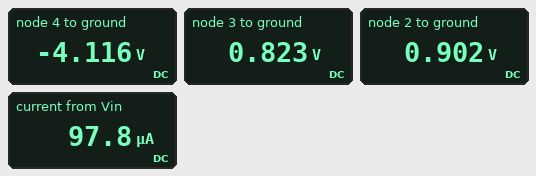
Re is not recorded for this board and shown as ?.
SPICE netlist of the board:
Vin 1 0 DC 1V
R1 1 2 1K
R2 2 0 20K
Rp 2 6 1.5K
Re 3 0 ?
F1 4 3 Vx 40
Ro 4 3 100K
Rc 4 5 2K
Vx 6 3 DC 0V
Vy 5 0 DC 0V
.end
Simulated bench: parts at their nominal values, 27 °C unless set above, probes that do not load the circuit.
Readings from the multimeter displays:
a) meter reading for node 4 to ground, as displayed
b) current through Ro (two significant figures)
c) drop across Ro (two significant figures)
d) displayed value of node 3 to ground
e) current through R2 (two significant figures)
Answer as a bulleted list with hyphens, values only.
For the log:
- -4.116 V
- 49 µA
- 4.9 V
- 0.823 V
- 45 µA
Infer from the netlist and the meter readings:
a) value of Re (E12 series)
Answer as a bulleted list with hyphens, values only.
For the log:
- 390 Ω
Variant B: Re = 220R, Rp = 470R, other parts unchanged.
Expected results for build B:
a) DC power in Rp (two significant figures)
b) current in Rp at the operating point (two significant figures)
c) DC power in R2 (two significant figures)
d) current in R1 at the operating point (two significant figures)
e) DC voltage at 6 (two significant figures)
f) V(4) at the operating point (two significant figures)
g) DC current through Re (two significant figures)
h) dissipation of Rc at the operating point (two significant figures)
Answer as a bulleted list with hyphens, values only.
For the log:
- 4.1 µW
- 93 µA
- 37 µW
- 140 µA
- 820 mV
- -7.3 V
- 3.7 mA
- 26 mW
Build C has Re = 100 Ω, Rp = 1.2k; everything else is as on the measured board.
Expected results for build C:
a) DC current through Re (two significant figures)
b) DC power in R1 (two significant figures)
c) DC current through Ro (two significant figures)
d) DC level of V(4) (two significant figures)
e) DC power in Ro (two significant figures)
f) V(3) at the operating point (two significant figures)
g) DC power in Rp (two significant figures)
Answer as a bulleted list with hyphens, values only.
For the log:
- 6.2 mA
- 38 µW
- 130 µA
- -12 V
- 1.6 mW
- 620 mV
- 29 µW
